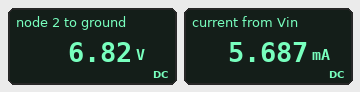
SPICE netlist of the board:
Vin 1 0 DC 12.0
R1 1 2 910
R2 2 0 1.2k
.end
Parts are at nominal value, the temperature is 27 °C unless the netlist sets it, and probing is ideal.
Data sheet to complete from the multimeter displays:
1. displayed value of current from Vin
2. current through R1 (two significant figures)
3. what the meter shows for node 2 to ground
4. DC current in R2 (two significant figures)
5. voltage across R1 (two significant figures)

5.687 mA
5.7 mA
6.82 V
5.7 mA
5.2 V
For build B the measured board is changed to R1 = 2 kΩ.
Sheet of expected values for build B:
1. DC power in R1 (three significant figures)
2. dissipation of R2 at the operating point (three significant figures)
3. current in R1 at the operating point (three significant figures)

28.1 mW
16.9 mW
3.75 mA
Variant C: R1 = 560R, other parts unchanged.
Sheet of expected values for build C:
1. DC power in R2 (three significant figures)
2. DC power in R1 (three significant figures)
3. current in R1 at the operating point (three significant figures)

55.8 mW
26.0 mW
6.82 mA
